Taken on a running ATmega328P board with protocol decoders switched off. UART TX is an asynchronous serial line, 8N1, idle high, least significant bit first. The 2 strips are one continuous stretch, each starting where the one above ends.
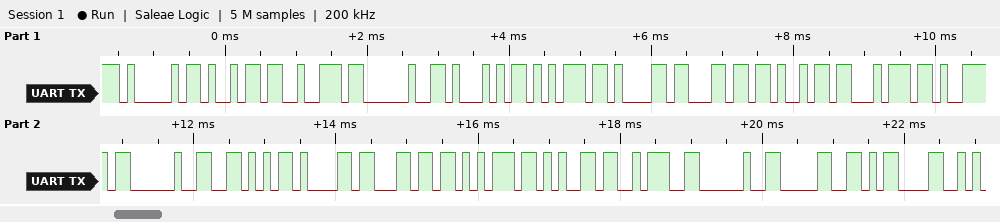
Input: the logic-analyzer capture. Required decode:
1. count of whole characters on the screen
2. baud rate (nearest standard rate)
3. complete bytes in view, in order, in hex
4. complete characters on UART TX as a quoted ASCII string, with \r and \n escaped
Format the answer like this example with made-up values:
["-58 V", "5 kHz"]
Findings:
["21", "9600 baud", "41 69 72 20 51 75 61 6C 69 74 79 20 56 61 6C 75 65 3A 20 30 0D", "\"Air Quality Value: 0\\r\""]
